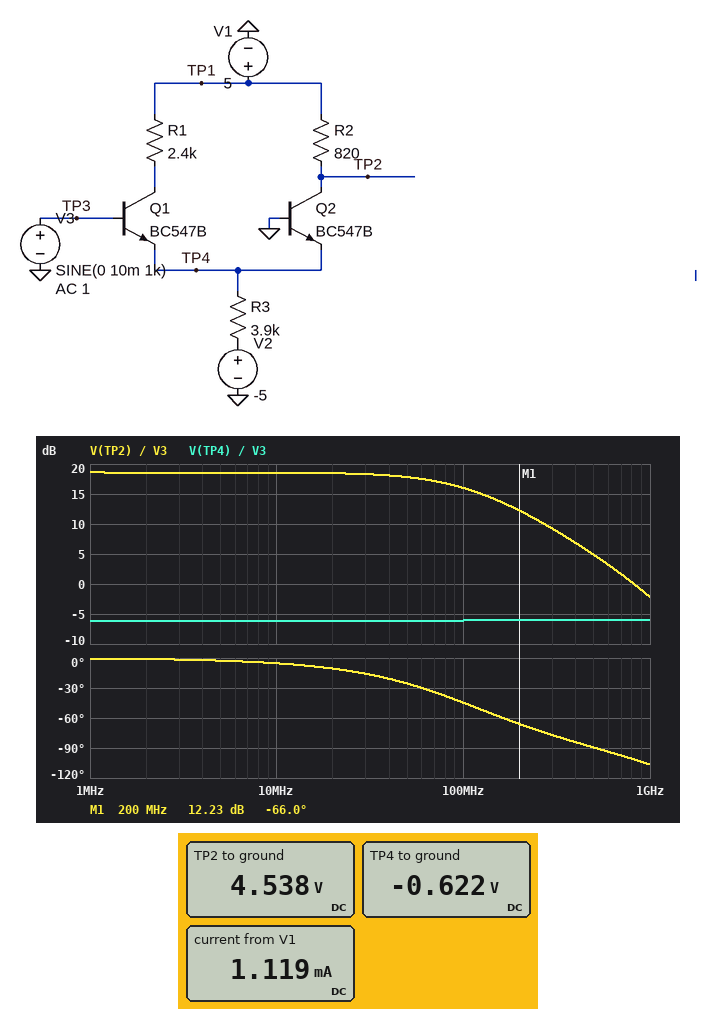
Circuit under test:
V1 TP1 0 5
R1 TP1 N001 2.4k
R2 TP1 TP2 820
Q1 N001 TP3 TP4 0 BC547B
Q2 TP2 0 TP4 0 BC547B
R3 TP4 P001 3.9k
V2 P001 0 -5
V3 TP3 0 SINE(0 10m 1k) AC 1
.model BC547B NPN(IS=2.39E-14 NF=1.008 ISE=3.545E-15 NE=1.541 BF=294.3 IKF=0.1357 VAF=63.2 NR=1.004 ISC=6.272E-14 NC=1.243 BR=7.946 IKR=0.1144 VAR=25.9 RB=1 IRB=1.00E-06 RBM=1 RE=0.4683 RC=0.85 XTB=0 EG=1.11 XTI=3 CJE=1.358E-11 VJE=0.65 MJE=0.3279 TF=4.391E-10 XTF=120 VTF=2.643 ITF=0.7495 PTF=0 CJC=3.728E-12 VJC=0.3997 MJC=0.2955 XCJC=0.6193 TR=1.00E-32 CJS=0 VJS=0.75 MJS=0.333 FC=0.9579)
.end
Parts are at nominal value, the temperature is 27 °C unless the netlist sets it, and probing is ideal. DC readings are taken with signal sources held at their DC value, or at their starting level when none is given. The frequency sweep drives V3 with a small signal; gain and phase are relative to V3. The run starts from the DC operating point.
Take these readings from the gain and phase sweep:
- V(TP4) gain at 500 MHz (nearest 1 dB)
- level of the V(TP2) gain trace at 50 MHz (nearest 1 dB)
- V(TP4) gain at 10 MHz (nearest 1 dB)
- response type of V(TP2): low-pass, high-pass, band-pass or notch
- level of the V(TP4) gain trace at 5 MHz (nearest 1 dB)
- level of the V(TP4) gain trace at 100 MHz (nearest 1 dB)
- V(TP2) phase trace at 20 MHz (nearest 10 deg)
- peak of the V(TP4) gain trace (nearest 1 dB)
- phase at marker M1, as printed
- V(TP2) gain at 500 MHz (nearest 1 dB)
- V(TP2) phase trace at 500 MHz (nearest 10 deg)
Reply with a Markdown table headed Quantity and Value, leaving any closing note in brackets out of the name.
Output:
| Quantity | Value |
|---|---|
| V(TP4) gain at 500 MHz | -6 dB |
| level of the V(TP2) gain trace at 50 MHz | 18 dB |
| V(TP4) gain at 10 MHz | -6 dB |
| response type of V(TP2): low-pass, high-pass, band-pass or notch | low-pass |
| level of the V(TP4) gain trace at 5 MHz | -6 dB |
| level of the V(TP4) gain trace at 100 MHz | -6 dB |
| V(TP2) phase trace at 20 MHz | -10 deg |
| peak of the V(TP4) gain trace | -6 dB |
| phase at marker M1, as printed | -66.0 deg |
| V(TP2) gain at 500 MHz | 5 dB |
| V(TP2) phase trace at 500 MHz | -90 deg |
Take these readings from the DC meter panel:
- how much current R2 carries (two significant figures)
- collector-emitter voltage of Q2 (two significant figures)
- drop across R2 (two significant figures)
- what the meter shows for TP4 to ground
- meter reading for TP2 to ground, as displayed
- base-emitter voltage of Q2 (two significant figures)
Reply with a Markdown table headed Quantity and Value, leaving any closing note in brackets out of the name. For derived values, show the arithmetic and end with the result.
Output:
| Quantity | Value |
|---|---|
| how much current R2 carries | (5 V - 4.538 V) / 820 Ω = 560 µA |
| collector-emitter voltage of Q2 | 4.538 V - (-622 mV) = 5.2 V |
| drop across R2 | 5 V - 4.538 V = 460 mV |
| what the meter shows for TP4 to ground | -0.622 V |
| meter reading for TP2 to ground, as displayed | 4.538 V |
| base-emitter voltage of Q2 | 0 V - (-622 mV) = 620 mV |
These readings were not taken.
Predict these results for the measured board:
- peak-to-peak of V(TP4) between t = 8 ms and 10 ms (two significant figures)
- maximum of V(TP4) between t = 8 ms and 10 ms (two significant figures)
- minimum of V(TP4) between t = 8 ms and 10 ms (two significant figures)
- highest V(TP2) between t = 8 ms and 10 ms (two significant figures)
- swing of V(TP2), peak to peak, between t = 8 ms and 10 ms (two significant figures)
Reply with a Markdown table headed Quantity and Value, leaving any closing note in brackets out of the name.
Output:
| Quantity | Value |
|---|---|
| peak-to-peak of V(TP4) between t = 8 ms and 10 ms | 9.8 mV |
| maximum of V(TP4) between t = 8 ms and 10 ms | -620 mV |
| minimum of V(TP4) between t = 8 ms and 10 ms | -630 mV |
| highest V(TP2) between t = 8 ms and 10 ms | 4.6 V |
| swing of V(TP2), peak to peak, between t = 8 ms and 10 ms | 170 mV |
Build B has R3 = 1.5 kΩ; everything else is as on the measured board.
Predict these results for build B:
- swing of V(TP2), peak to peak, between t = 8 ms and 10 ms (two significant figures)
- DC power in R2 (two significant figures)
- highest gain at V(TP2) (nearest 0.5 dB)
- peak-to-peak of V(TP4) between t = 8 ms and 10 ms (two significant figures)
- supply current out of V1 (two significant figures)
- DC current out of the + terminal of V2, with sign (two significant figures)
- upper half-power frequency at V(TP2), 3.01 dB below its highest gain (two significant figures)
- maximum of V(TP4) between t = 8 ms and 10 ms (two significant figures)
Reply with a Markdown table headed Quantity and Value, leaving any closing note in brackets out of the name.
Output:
| Quantity | Value |
|---|---|
| swing of V(TP2), peak to peak, between t = 8 ms and 10 ms | 420 mV |
| DC power in R2 | 1.8 mW |
| highest gain at V(TP2) | 26.5 dB |
| peak-to-peak of V(TP4) between t = 8 ms and 10 ms | 9.6 mV |
| supply current out of V1 | 2.9 mA |
| DC current out of the + terminal of V2, with sign | -2.9 mA |
| upper half-power frequency at V(TP2), 3.01 dB below its highest gain | 110 MHz |
| maximum of V(TP4) between t = 8 ms and 10 ms | -640 mV |
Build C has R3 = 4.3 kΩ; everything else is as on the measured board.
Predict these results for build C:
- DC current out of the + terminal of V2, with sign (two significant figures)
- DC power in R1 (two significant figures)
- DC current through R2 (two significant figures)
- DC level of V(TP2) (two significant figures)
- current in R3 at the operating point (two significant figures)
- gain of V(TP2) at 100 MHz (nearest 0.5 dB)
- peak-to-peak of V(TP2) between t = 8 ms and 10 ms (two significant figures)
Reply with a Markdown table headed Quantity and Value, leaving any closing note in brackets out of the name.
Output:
| Quantity | Value |
|---|---|
| DC current out of the + terminal of V2, with sign | -1.0 mA |
| DC power in R1 | 610 µW |
| DC current through R2 | 510 µA |
| DC level of V(TP2) | 4.6 V |
| current in R3 at the operating point | 1.0 mA |
| gain of V(TP2) at 100 MHz | 15.0 dB |
| peak-to-peak of V(TP2) between t = 8 ms and 10 ms | 150 mV |
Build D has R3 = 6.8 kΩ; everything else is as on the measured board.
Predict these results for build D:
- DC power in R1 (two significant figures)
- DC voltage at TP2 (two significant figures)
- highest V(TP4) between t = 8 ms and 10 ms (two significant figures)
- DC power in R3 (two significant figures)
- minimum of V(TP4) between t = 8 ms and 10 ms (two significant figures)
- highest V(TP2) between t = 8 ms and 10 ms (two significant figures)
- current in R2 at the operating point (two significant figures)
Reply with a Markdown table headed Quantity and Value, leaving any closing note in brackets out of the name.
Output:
| Quantity | Value |
|---|---|
| DC power in R1 | 250 µW |
| DC voltage at TP2 | 4.7 V |
| highest V(TP4) between t = 8 ms and 10 ms | -600 mV |
| DC power in R3 | 2.8 mW |
| minimum of V(TP4) between t = 8 ms and 10 ms | -610 mV |
| highest V(TP2) between t = 8 ms and 10 ms | 4.8 V |
| current in R2 at the operating point | 320 µA |
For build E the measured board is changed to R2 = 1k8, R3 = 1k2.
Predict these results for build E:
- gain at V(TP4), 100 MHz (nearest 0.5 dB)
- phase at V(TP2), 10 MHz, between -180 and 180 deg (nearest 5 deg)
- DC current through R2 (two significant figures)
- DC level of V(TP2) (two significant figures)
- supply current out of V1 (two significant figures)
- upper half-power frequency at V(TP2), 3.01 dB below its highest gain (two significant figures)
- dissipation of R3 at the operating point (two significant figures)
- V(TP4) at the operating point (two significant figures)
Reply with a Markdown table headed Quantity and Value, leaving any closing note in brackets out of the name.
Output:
| Quantity | Value |
|---|---|
| gain at V(TP4), 100 MHz | -6.0 dB |
| phase at V(TP2), 10 MHz, between -180 and 180 deg | -15 deg |
| DC current through R2 | 1.8 mA |
| DC level of V(TP2) | 1.7 V |
| supply current out of V1 | 3.6 mA |
| upper half-power frequency at V(TP2), 3.01 dB below its highest gain | 40 MHz |
| dissipation of R3 at the operating point | 16 mW |
| V(TP4) at the operating point | -650 mV |
